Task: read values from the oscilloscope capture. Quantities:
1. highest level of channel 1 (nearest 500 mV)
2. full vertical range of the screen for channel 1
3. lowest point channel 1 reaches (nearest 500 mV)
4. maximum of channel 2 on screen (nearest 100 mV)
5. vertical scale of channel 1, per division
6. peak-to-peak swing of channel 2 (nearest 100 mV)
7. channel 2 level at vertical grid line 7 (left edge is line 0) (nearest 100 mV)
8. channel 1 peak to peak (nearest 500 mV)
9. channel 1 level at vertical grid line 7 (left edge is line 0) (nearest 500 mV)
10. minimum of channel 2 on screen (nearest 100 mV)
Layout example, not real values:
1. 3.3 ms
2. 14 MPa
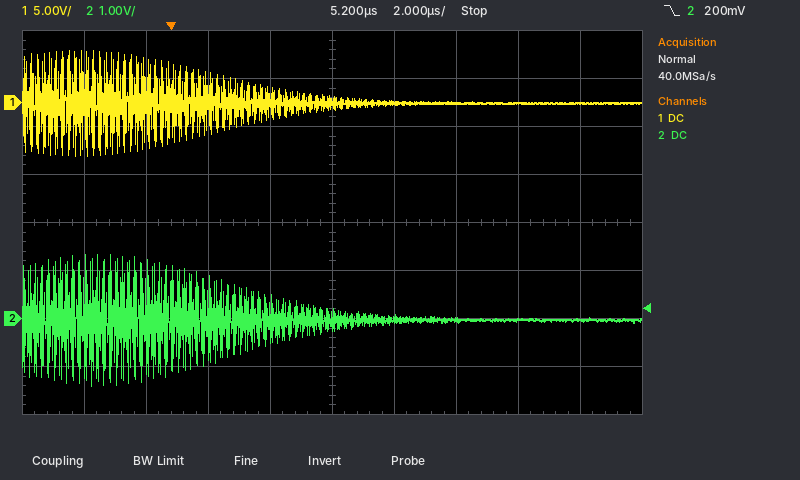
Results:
1. 5.5 V
2. 40 V
3. -5.5 V
4. 1.3 V
5. 5 V
6. 2.7 V
7. 0.0 V
8. 11.0 V
9. 0.0 V
10. -1.4 V
